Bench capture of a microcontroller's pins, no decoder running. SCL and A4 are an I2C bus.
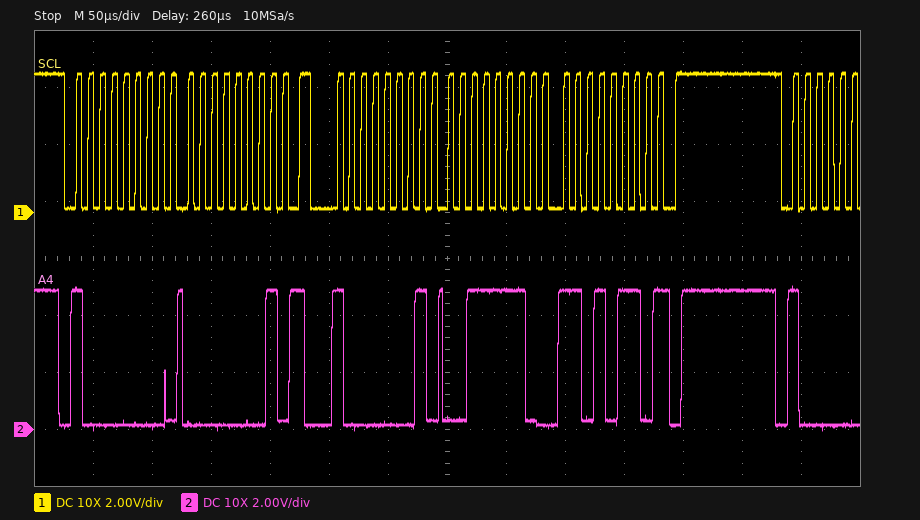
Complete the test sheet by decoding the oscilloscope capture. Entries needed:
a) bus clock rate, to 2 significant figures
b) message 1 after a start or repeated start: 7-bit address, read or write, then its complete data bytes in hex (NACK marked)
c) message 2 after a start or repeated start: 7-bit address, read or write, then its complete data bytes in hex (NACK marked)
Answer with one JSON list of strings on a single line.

["100 kHz", "0x40 write: 01", "0x40 read: 3E D6 NACK"]
